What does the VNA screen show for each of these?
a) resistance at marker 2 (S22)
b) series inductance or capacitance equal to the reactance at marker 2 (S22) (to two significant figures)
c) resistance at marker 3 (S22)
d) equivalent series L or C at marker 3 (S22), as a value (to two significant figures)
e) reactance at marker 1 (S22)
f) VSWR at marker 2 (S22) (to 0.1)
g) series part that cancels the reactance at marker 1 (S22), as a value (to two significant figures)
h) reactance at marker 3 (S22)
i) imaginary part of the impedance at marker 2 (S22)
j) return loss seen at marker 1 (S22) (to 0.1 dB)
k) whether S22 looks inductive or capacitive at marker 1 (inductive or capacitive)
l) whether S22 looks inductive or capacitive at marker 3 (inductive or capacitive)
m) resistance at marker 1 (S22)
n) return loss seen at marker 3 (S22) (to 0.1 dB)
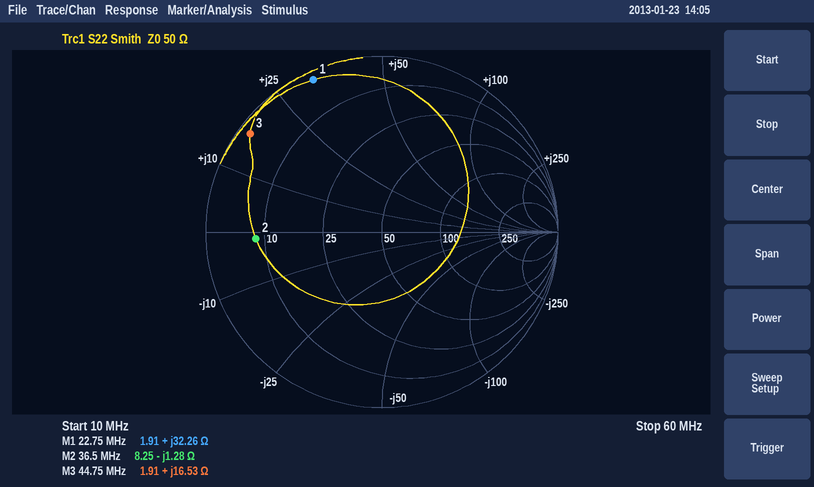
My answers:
8.25 Ω
3.4 nF
1.91 Ω
59 nH
+32.26 Ω
6.1
220 pF
+16.53 Ω
-1.28 Ω
0.5 dB
inductive
inductive
1.91 Ω
0.6 dB
